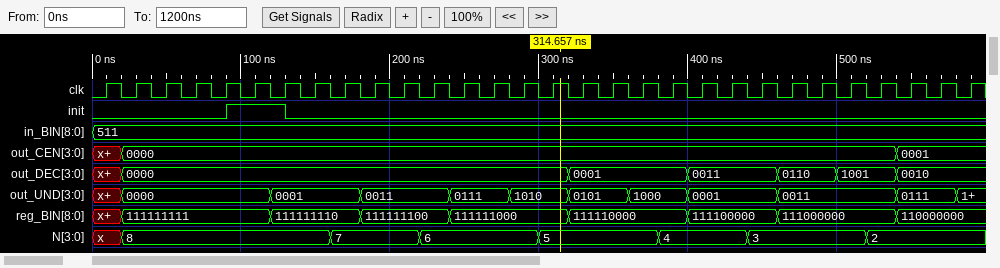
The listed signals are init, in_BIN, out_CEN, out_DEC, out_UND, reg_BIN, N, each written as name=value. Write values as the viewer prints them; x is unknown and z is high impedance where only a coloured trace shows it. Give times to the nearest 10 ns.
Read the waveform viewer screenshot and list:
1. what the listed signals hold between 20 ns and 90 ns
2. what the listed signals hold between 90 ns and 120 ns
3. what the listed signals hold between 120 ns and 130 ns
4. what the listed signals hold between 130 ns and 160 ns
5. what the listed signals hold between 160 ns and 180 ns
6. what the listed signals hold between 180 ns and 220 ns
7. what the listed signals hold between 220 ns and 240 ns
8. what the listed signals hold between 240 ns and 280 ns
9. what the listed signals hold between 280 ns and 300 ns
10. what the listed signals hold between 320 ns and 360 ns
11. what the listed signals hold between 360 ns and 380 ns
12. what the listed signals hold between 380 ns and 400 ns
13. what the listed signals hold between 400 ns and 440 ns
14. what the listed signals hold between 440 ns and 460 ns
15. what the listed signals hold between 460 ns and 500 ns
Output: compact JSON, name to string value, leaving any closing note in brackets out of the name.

{"what the listed signals hold between 20 ns and 90 ns": "init=0, in_BIN=511, out_CEN=0000, out_DEC=0000, out_UND=0000, reg_BIN=111111111, N=8", "what the listed signals hold between 90 ns and 120 ns": "init=1, in_BIN=511, out_CEN=0000, out_DEC=0000, out_UND=0000, reg_BIN=111111111, N=8", "what the listed signals hold between 120 ns and 130 ns": "init=1, in_BIN=511, out_CEN=0000, out_DEC=0000, out_UND=0001, reg_BIN=111111110, N=8", "what the listed signals hold between 130 ns and 160 ns": "init=0, in_BIN=511, out_CEN=0000, out_DEC=0000, out_UND=0001, reg_BIN=111111110, N=8", "what the listed signals hold between 160 ns and 180 ns": "init=0, in_BIN=511, out_CEN=0000, out_DEC=0000, out_UND=0001, reg_BIN=111111110, N=7", "what the listed signals hold between 180 ns and 220 ns": "init=0, in_BIN=511, out_CEN=0000, out_DEC=0000, out_UND=0011, reg_BIN=111111100, N=7", "what the listed signals hold between 220 ns and 240 ns": "init=0, in_BIN=511, out_CEN=0000, out_DEC=0000, out_UND=0011, reg_BIN=111111100, N=6", "what the listed signals hold between 240 ns and 280 ns": "init=0, in_BIN=511, out_CEN=0000, out_DEC=0000, out_UND=0111, reg_BIN=111111000, N=6", "what the listed signals hold between 280 ns and 300 ns": "init=0, in_BIN=511, out_CEN=0000, out_DEC=0000, out_UND=1010, reg_BIN=111111000, N=6", "what the listed signals hold between 320 ns and 360 ns": "init=0, in_BIN=511, out_CEN=0000, out_DEC=0001, out_UND=0101, reg_BIN=111110000, N=5", "what the listed signals hold between 360 ns and 380 ns": "init=0, in_BIN=511, out_CEN=0000, out_DEC=0001, out_UND=1000, reg_BIN=111110000, N=5", "what the listed signals hold between 380 ns and 400 ns": "init=0, in_BIN=511, out_CEN=0000, out_DEC=0001, out_UND=1000, reg_BIN=111110000, N=4", "what the listed signals hold between 400 ns and 440 ns": "init=0, in_BIN=511, out_CEN=0000, out_DEC=0011, out_UND=0001, reg_BIN=111100000, N=4", "what the listed signals hold between 440 ns and 460 ns": "init=0, in_BIN=511, out_CEN=0000, out_DEC=0011, out_UND=0001, reg_BIN=111100000, N=3", "what the listed signals hold between 460 ns and 500 ns": "init=0, in_BIN=511, out_CEN=0000, out_DEC=0110, out_UND=0011, reg_BIN=111000000, N=3"}
